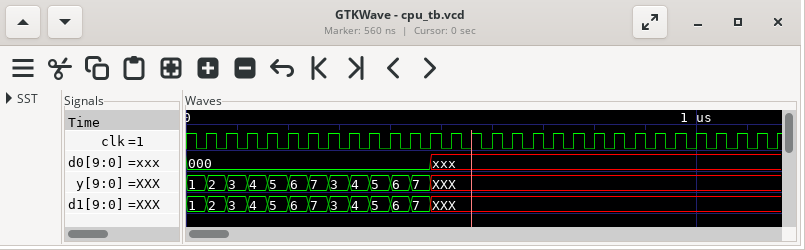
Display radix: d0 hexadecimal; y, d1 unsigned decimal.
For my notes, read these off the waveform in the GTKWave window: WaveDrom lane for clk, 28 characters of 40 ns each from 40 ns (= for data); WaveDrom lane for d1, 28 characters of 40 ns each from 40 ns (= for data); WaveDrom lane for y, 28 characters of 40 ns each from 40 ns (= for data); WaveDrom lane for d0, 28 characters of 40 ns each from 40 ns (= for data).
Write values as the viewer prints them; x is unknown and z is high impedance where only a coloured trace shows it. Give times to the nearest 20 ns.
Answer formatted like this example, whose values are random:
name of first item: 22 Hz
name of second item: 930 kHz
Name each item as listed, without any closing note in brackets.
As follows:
WaveDrom lane for clk, 28 characters of 40 ns each from 40 ns: {name: 'clk', wave: 'p...........................'}
WaveDrom lane for d1, 28 characters of 40 ns each from 40 ns: {name: 'd1', wave: '===========x................', data: '2 3 4 5 6 7 3 4 5 6 7'}
WaveDrom lane for y, 28 characters of 40 ns each from 40 ns: {name: 'y', wave: '===========x................', data: '2 3 4 5 6 7 3 4 5 6 7'}
WaveDrom lane for d0, 28 characters of 40 ns each from 40 ns: {name: 'd0', wave: '=..........x................', data: '000'}
